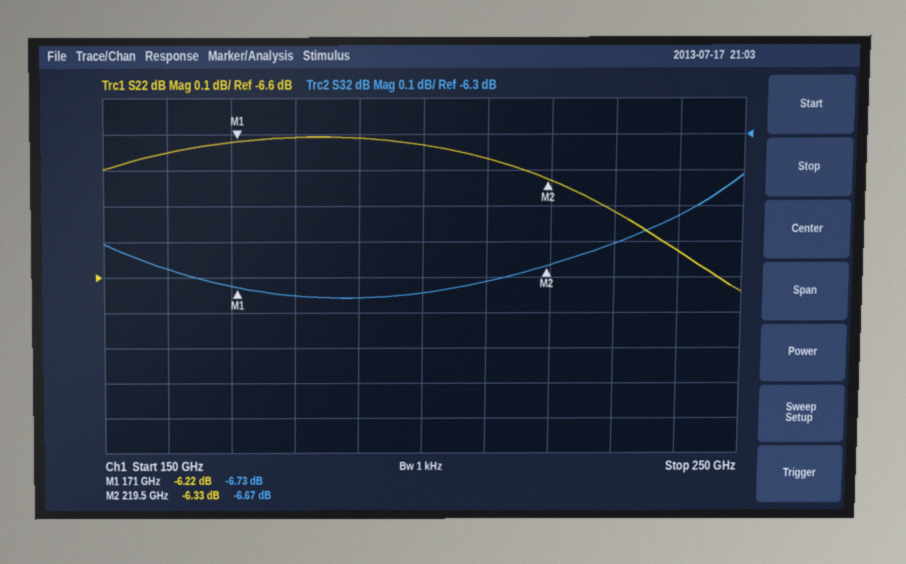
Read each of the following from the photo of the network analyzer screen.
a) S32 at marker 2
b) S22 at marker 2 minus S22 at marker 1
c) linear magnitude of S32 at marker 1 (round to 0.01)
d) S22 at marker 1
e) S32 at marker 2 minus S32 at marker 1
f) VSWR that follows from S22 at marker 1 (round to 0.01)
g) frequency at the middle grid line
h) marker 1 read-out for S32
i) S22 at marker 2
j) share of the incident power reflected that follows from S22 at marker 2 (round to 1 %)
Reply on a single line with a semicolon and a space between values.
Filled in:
-6.67 dB; -0.11 dB; 0.46; -6.22 dB; 0.06 dB; 2.91; 200 GHz; -6.73 dB; -6.33 dB; 23 %
